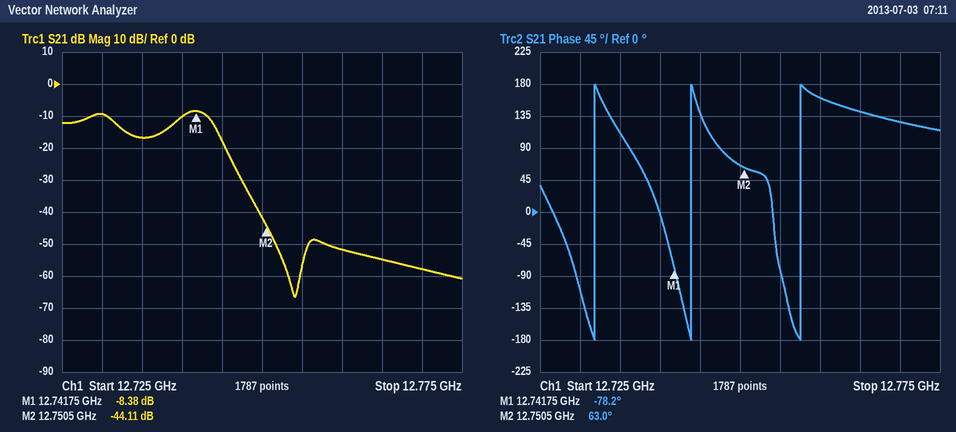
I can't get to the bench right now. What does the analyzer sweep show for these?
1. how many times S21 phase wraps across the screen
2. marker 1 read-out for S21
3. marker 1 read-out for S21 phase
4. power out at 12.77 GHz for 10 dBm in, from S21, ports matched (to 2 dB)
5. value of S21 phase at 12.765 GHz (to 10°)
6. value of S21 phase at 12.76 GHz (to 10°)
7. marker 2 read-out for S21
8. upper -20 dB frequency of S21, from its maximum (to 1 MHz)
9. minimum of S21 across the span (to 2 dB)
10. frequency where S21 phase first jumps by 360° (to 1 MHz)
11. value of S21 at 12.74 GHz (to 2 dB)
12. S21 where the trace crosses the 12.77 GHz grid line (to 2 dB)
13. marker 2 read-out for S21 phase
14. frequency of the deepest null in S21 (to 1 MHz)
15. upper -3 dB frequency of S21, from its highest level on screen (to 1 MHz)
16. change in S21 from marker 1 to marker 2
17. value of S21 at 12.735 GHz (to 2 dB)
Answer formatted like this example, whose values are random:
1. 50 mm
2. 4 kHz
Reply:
1. 3
2. -8.38 dB
3. -78.2°
4. -48 dBm
5. 140°
6. 160°
7. -44.11 dB
8. 12.747 GHz
9. -66 dB
10. 12.732 GHz
11. -10 dB
12. -58 dB
13. 63.0°
14. 12.754 GHz
15. 12.744 GHz
16. -35.73 dB
17. -16 dB
